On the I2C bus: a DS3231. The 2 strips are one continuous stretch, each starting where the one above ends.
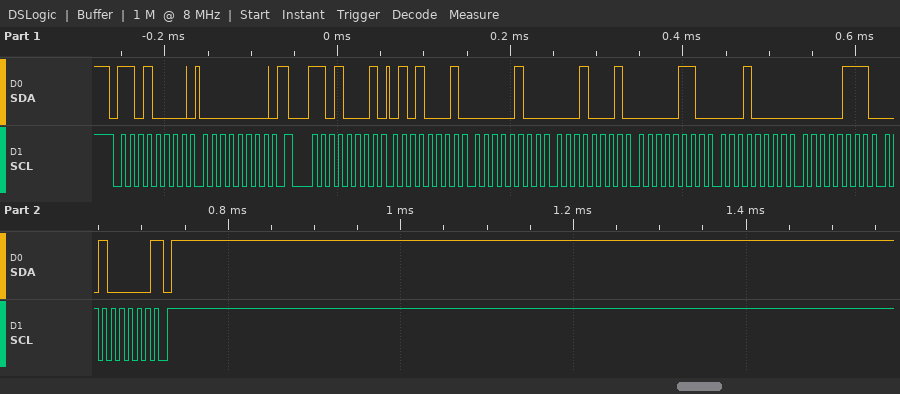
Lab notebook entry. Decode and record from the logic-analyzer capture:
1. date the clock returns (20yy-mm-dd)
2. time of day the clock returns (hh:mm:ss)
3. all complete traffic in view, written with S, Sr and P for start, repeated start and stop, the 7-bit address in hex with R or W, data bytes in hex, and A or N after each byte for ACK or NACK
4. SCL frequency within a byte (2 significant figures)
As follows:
2020-07-10
11:04:51
S 68W A 00 A Sr 68R A 51 A 04 A 11 A 06 A 10 A 07 A 20 N P
100 kHz
